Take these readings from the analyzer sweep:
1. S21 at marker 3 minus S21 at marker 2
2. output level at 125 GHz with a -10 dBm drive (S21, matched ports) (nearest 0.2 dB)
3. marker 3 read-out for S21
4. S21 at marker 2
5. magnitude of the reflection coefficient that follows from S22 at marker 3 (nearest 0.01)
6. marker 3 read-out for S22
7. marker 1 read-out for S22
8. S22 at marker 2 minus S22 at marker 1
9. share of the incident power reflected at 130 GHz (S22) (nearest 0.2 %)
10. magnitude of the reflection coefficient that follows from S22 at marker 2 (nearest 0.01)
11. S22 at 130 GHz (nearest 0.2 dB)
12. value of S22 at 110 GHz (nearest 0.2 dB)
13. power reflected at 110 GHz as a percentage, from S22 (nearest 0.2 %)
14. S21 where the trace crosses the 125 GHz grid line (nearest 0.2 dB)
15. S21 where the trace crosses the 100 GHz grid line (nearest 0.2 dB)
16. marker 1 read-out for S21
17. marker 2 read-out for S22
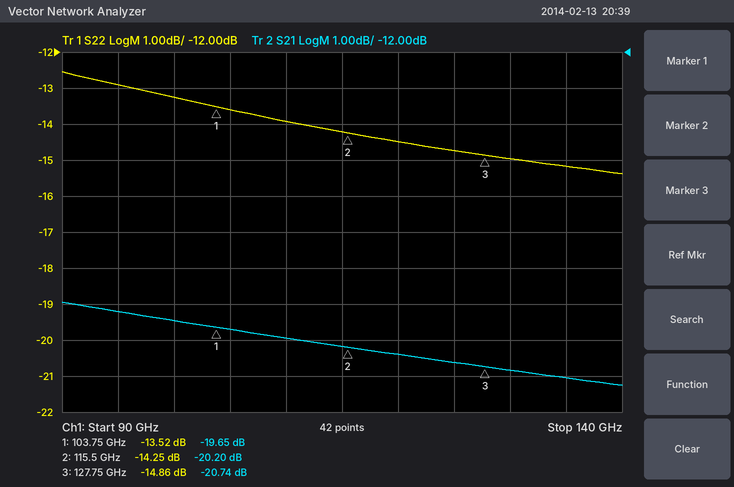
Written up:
-0.54 dB
-30.6 dBm
-20.74 dB
-20.20 dB
0.18
-14.86 dB
-13.52 dB
-0.73 dB
3.2 %
0.19
-15.0 dB
-14.0 dB
4.0 %
-20.6 dB
-19.4 dB
-19.65 dB
-14.25 dB
